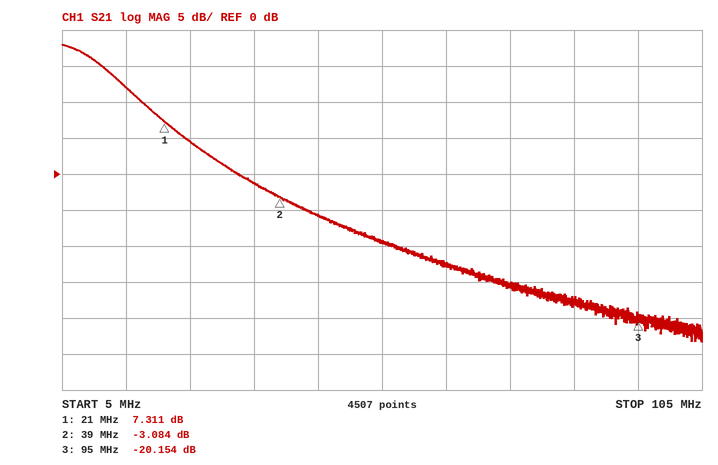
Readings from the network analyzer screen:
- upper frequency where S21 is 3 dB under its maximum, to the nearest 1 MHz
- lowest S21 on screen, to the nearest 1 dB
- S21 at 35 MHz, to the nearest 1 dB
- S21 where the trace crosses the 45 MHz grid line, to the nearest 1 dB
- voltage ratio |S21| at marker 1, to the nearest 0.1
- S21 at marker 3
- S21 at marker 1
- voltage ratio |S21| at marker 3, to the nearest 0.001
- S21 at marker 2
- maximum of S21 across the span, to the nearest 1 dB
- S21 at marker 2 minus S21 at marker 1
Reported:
11 MHz
-23 dB
-1 dB
-6 dB
2.3
-20.154 dB
7.311 dB
0.098
-3.084 dB
18 dB
-10.395 dB
